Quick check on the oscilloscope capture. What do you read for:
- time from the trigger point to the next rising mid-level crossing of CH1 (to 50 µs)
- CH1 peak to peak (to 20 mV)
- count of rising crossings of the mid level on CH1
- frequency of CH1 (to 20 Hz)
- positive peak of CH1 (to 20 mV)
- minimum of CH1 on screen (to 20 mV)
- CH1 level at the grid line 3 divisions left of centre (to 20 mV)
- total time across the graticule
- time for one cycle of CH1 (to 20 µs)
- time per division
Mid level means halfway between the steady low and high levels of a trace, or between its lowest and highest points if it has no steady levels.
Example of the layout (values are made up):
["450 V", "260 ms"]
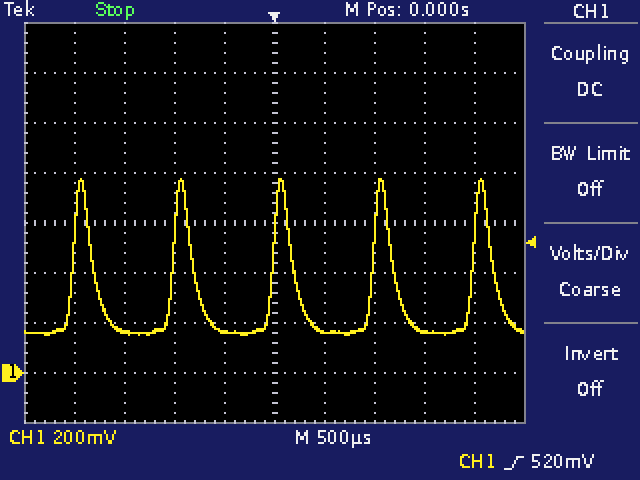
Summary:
["1.00 ms", "620 mV", "5", "1.00 kHz", "780 mV", "160 mV", "160 mV", "5 ms", "1.00 ms", "500 µs"]
